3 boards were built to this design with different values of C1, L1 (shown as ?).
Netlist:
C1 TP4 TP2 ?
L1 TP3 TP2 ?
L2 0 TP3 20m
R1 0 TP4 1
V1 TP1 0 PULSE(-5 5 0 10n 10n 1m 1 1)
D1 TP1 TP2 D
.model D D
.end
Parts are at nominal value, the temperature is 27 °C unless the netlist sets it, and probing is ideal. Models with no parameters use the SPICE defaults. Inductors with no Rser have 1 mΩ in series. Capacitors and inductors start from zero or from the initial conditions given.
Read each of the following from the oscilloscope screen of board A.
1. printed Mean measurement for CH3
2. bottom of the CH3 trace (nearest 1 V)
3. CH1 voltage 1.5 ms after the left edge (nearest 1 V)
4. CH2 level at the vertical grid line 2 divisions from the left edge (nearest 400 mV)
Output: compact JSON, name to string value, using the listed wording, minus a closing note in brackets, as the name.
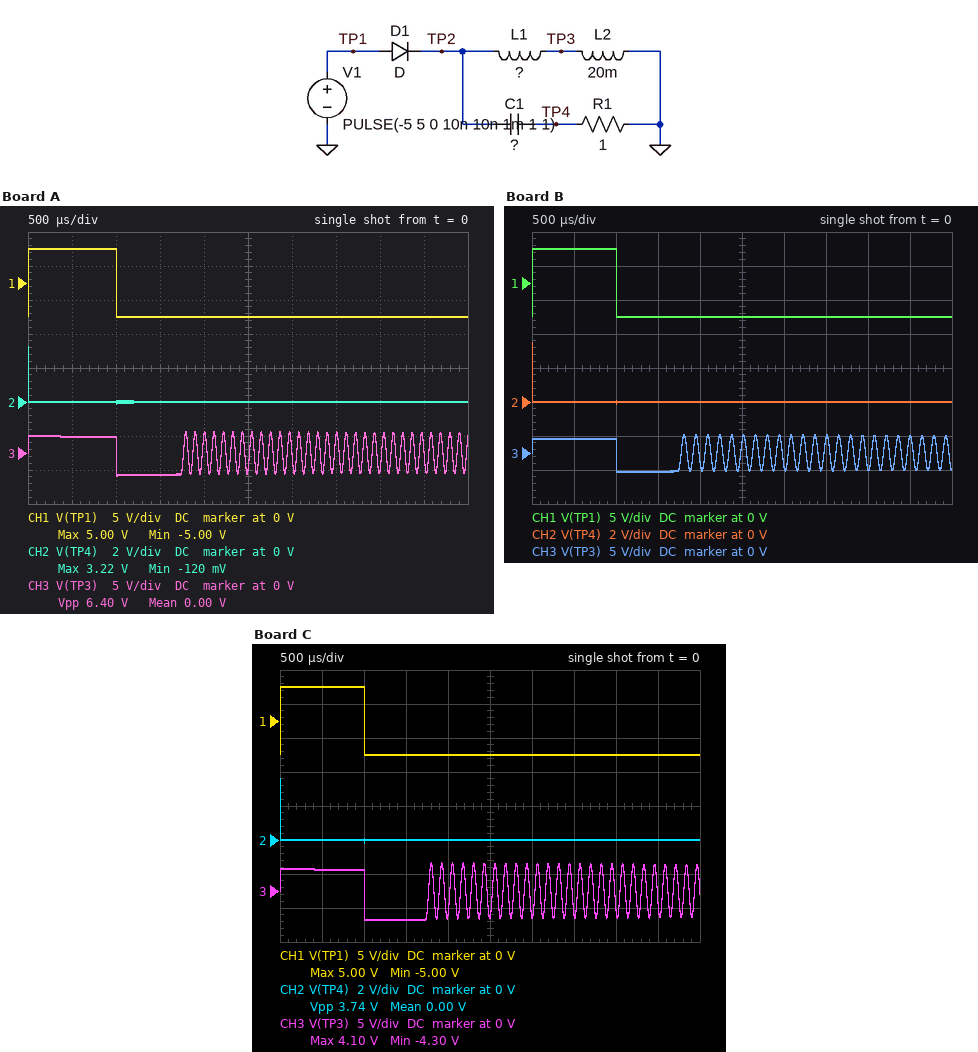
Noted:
{"printed Mean measurement for CH3": "0.00 V", "bottom of the CH3 trace": "-3 V", "CH1 voltage 1.5 ms after the left edge": "-5 V", "CH2 level at the vertical grid line 2 divisions from the left edge": "0 V"}
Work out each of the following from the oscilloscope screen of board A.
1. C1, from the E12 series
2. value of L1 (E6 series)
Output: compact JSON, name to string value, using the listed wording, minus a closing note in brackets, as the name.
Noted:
{"C1, from the E12 series": "8.2 nF", "value of L1": "15 mH"}
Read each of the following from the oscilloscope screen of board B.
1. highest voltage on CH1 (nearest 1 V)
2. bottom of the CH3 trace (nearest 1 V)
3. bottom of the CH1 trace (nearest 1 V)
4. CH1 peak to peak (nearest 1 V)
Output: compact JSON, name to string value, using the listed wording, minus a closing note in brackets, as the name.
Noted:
{"highest voltage on CH1": "5 V", "bottom of the CH3 trace": "-3 V", "bottom of the CH1 trace": "-5 V", "CH1 peak to peak": "10 V"}
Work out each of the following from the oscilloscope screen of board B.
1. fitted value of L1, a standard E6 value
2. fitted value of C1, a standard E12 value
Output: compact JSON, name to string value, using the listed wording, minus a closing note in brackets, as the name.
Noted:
{"fitted value of L1, a standard E6 value": "22 mH", "fitted value of C1, a standard E12 value": "12 nF"}
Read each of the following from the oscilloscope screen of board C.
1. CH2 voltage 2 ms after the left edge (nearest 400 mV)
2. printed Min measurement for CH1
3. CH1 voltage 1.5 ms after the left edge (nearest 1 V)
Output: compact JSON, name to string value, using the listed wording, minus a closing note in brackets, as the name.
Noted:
{"CH2 voltage 2 ms after the left edge": "0 V", "printed Min measurement for CH1": "-5.00 V", "CH1 voltage 1.5 ms after the left edge": "-5 V"}
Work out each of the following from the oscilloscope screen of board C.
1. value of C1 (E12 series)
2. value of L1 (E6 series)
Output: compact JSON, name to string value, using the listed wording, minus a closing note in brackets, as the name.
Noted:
{"value of C1": "15 nF", "value of L1": "6.8 mH"}
